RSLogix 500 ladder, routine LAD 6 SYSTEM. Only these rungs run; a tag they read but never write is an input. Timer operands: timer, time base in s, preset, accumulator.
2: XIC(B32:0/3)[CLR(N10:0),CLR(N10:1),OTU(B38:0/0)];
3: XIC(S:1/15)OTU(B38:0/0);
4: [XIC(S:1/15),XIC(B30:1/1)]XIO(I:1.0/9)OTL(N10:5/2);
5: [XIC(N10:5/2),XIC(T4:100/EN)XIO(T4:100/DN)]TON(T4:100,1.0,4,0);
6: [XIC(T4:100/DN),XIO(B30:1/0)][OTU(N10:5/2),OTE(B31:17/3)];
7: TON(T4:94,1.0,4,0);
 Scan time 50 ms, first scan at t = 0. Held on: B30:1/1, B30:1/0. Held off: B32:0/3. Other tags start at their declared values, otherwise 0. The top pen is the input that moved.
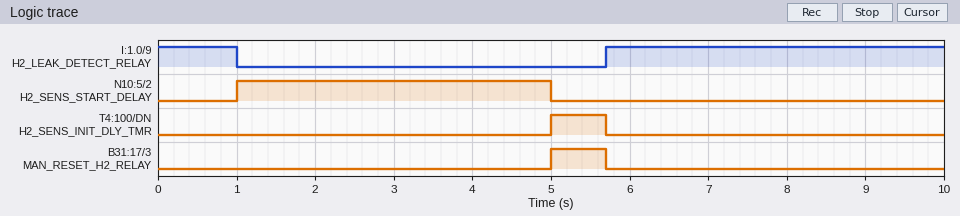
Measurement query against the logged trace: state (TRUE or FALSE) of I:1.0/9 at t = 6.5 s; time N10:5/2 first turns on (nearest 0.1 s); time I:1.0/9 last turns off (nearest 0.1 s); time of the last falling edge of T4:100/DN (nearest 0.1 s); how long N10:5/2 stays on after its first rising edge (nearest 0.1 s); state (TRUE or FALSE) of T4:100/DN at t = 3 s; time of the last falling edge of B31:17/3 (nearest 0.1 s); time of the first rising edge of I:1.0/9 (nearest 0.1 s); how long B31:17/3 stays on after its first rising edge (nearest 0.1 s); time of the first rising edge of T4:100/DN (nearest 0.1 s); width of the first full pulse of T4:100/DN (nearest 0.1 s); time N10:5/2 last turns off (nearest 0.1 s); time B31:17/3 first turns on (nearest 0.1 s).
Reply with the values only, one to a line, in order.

TRUE
1.0 s
1.0 s
5.7 s
4.0 s
FALSE
5.7 s
5.7 s
0.7 s
5.0 s
0.7 s
5.0 s
5.0 s
